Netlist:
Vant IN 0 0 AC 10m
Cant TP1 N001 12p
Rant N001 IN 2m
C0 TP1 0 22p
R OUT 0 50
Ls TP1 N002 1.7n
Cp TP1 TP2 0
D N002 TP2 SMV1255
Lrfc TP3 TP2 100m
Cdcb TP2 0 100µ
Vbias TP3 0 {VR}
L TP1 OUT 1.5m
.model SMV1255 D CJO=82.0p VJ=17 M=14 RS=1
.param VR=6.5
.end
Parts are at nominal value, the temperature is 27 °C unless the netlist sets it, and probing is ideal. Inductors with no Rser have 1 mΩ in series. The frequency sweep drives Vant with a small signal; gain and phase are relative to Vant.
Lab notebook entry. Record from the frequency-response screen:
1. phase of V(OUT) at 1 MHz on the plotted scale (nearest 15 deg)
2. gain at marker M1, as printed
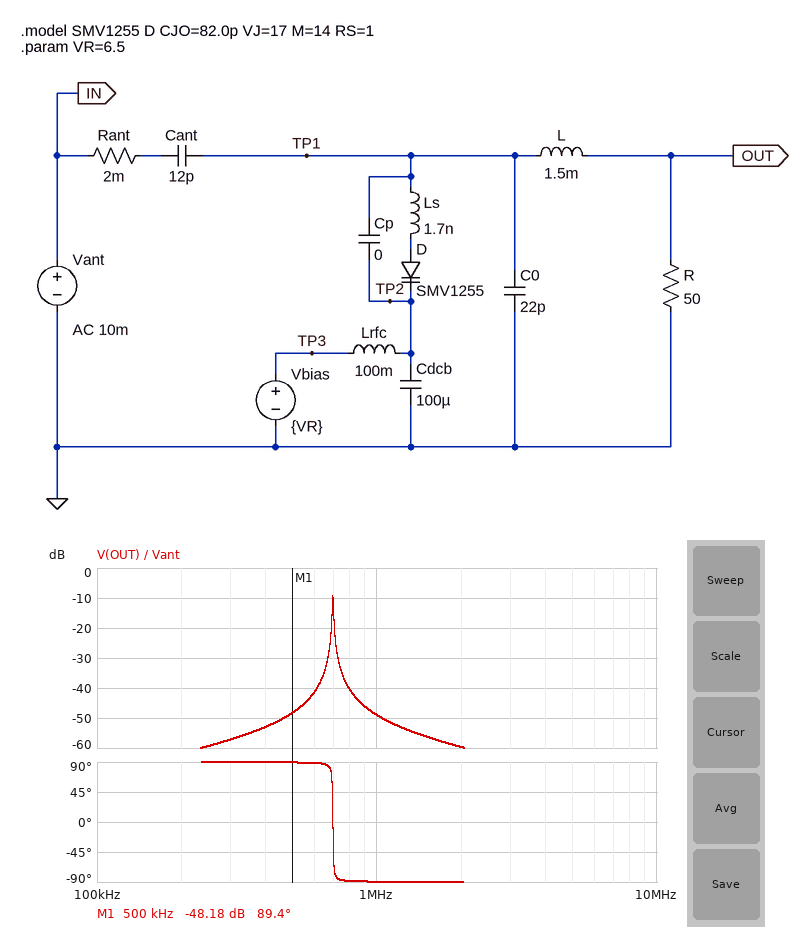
-90 deg
-48.18 dB
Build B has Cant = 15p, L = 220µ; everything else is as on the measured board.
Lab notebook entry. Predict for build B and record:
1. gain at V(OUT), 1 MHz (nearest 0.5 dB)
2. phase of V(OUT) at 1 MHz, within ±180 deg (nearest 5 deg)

-43.0 dB
90 deg
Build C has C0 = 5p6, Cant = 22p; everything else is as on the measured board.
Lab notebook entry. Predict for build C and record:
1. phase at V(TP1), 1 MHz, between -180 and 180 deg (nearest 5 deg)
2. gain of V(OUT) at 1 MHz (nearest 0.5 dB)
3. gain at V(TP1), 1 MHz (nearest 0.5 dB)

0 deg
-40.0 dB
5.5 dB
